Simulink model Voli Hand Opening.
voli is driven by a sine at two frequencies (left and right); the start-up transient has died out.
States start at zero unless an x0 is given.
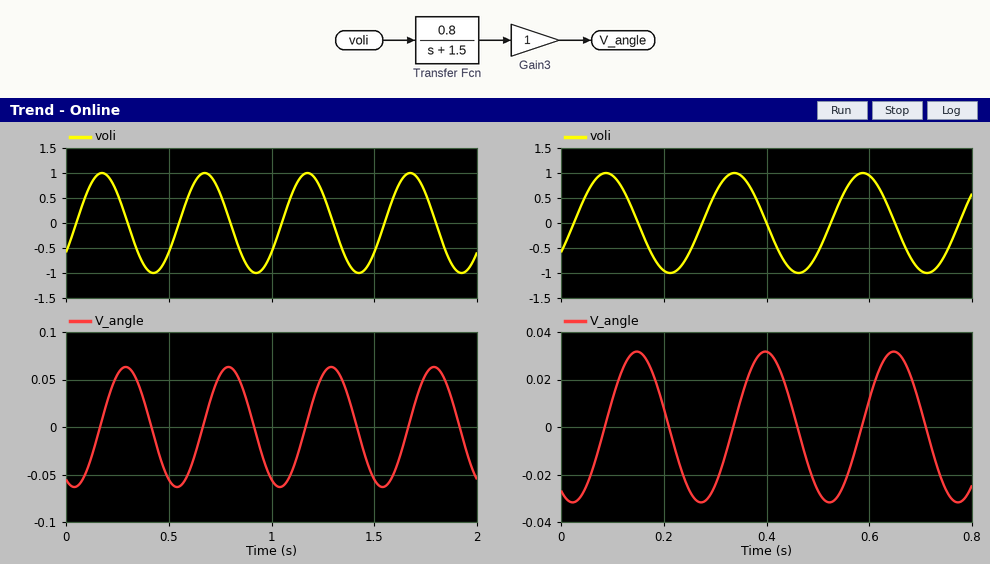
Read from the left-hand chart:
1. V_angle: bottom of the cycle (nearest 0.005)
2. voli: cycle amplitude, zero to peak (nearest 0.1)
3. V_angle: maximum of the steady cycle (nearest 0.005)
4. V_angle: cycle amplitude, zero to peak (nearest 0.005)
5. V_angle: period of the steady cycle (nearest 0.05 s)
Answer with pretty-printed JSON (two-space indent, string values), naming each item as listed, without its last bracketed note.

{
  "V_angle: bottom of the cycle": "-0.065",
  "voli: cycle amplitude, zero to peak": "1.0",
  "V_angle: maximum of the steady cycle": "0.065",
  "V_angle: cycle amplitude, zero to peak": "0.065",
  "V_angle: period of the steady cycle": "0.50 s"
}
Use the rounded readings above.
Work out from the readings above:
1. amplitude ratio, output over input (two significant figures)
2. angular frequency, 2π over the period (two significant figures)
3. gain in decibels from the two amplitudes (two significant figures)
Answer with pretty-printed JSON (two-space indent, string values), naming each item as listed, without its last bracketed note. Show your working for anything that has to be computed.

{
  "amplitude ratio, output over input": "0.065 / 1 = 0.065",
  "angular frequency, 2π over the period": "2π / 0.5 = 13 rad/s",
  "gain in decibels from the two amplitudes": "20 log10(0.065 / 1) = -24 dB"
}
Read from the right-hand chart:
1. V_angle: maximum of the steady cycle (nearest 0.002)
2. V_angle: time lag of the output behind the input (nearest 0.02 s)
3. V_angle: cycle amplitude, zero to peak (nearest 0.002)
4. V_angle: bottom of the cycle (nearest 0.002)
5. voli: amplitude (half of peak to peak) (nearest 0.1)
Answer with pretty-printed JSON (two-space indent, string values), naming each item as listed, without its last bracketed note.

{
  "V_angle: maximum of the steady cycle": "0.032",
  "V_angle: time lag of the output behind the input": "0.06 s",
  "V_angle: cycle amplitude, zero to peak": "0.032",
  "V_angle: bottom of the cycle": "-0.032",
  "voli: amplitude (half of peak to peak)": "1.0"
}
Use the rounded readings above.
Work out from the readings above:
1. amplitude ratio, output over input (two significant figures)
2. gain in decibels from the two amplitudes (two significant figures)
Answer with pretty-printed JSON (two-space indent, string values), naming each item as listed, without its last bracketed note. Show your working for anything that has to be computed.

{
  "amplitude ratio, output over input": "0.032 / 1 = 0.032",
  "gain in decibels from the two amplitudes": "20 log10(0.032 / 1) = -30 dB"
}
